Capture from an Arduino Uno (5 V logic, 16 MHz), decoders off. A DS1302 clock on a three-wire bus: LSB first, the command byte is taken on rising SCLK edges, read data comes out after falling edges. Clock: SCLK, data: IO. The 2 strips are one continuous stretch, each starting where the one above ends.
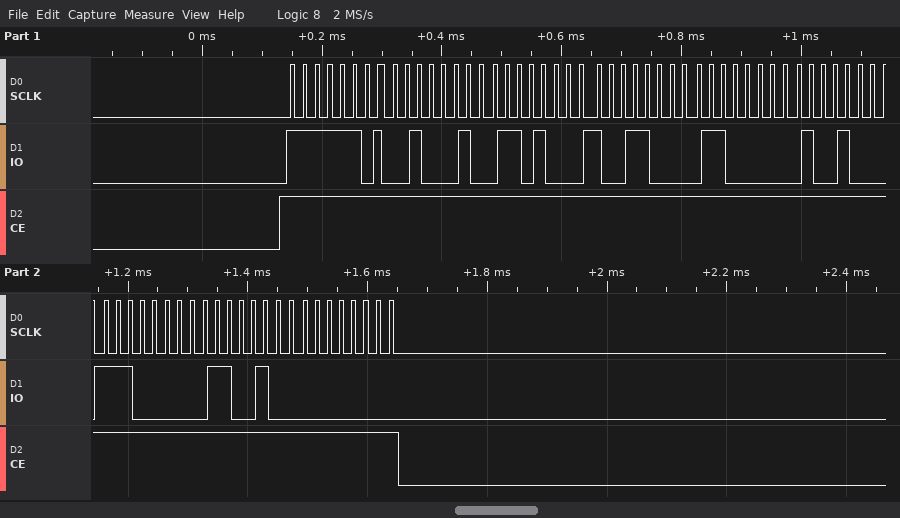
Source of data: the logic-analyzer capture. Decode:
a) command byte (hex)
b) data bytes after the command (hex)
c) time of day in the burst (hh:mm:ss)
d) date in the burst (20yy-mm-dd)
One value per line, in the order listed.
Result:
0xBF
44 16 19 06 12 07 26 00
19:16:44
2026-12-06
